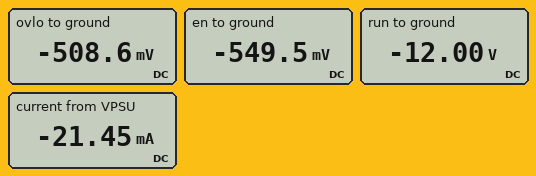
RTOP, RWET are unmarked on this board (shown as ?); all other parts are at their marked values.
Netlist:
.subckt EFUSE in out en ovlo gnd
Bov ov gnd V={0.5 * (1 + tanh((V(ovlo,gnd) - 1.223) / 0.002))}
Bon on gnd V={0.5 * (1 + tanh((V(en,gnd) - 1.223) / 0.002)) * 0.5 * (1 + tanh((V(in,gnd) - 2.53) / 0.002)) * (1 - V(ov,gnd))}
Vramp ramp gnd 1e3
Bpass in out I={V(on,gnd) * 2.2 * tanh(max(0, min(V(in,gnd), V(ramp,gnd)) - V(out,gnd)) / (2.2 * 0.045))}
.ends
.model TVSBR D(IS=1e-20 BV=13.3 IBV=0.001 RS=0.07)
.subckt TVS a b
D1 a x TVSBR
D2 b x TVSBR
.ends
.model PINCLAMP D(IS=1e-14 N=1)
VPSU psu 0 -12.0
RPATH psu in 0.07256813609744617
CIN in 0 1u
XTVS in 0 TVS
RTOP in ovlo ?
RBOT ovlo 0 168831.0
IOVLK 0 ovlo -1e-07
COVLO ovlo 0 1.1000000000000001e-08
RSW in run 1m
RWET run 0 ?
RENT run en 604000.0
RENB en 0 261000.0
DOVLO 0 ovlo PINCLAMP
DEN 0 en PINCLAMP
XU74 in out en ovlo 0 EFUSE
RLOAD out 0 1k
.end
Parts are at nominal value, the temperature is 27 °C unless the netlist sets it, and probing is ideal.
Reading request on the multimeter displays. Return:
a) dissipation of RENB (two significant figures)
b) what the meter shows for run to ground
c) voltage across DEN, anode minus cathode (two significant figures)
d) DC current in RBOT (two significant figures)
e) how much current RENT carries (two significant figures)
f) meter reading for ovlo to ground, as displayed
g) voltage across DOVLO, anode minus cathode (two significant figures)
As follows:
1.2 µW
-12.00 V
550 mV
3.0 µA
19 µA
-508.6 mV
510 mV
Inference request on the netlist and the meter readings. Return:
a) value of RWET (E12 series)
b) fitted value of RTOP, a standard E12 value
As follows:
560 Ω
1.8 MΩ
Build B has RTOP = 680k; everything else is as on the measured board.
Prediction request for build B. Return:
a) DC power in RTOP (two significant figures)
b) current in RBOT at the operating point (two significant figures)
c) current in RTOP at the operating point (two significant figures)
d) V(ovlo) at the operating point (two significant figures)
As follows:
190 µW
3.2 µA
17 µA
-540 mV
